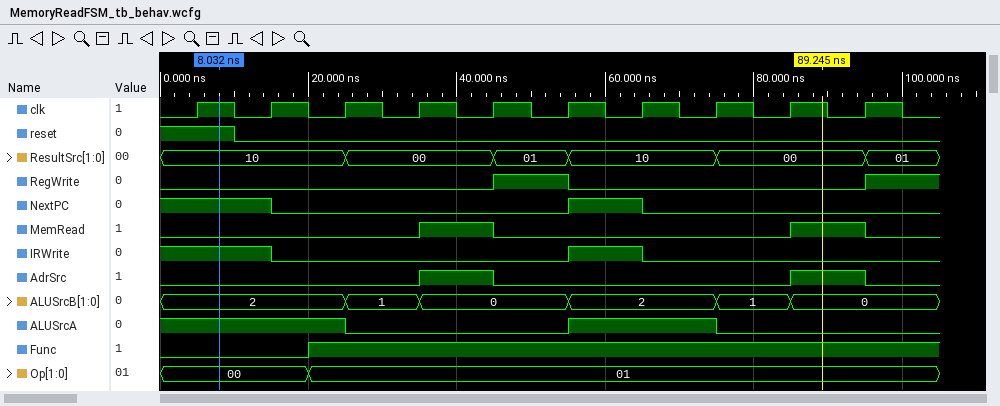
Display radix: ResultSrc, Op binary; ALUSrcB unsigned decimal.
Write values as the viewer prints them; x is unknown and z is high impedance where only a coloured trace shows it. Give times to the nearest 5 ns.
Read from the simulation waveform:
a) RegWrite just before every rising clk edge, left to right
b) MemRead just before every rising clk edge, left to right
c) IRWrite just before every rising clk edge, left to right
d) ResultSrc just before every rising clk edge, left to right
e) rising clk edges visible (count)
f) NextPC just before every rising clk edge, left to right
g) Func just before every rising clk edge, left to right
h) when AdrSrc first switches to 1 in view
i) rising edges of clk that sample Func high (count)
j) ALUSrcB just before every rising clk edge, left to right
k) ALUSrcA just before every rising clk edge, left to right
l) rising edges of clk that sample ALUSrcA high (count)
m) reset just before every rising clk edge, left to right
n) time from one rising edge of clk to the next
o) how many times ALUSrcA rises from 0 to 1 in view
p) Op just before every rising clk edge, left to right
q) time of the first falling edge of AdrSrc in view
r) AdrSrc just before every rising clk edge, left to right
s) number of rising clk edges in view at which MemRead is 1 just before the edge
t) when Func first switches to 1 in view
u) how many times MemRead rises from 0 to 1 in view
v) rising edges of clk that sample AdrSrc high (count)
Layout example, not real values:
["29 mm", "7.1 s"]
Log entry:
["0 0 0 0 0 1 0 0 0 0", "0 0 0 0 1 0 0 0 0 1", "1 1 0 0 0 0 1 0 0 0", "10, 10, 10, 00, 00, 01, 10, 10, 00, 00", "10", "1 1 0 0 0 0 1 0 0 0", "0 0 1 1 1 1 1 1 1 1", "35 ns", "8", "2, 2, 2, 1, 0, 0, 2, 2, 1, 0", "1 1 1 0 0 0 1 1 0 0", "5", "1 0 0 0 0 0 0 0 0 0", "10 ns", "1", "00, 00, 01, 01, 01, 01, 01, 01, 01, 01", "45 ns", "0 0 0 0 1 0 0 0 0 1", "2", "20 ns", "2", "2"]
